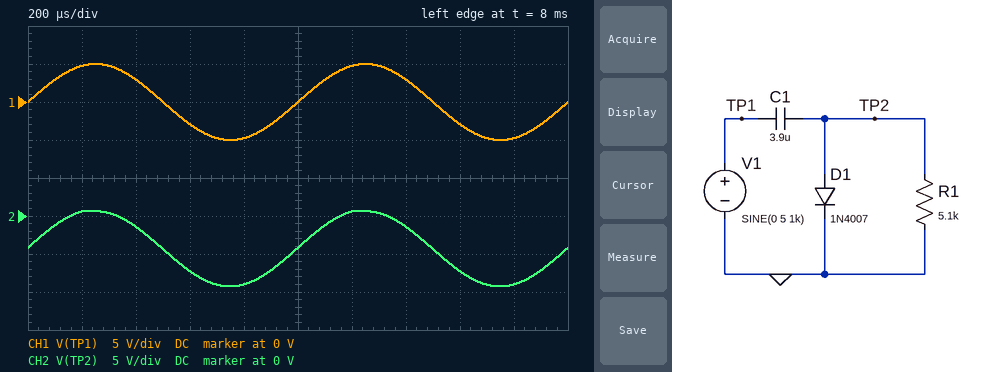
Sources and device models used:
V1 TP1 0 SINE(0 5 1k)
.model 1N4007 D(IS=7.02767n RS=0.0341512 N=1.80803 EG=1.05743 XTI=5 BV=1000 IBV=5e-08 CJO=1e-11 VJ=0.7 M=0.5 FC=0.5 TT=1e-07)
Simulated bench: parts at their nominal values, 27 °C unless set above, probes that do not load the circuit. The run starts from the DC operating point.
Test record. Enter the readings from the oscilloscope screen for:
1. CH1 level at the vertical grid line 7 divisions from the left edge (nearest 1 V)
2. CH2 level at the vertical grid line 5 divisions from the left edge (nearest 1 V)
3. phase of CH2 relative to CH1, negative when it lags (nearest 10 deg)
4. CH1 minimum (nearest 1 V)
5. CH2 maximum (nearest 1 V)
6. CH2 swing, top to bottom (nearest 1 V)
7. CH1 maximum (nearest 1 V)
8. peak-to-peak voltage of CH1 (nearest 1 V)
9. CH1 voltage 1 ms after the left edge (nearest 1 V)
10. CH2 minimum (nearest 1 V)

3 V
-4 V
0 deg
-5 V
1 V
10 V
5 V
10 V
0 V
-9 V
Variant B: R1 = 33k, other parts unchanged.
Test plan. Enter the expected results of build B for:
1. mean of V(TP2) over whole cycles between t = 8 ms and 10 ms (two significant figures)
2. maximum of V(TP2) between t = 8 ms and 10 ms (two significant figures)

-4.4 V
610 mV
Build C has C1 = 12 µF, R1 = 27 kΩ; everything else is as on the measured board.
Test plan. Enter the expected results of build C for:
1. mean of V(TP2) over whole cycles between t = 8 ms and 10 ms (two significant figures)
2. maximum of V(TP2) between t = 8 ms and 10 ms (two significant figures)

-4.4 V
630 mV
